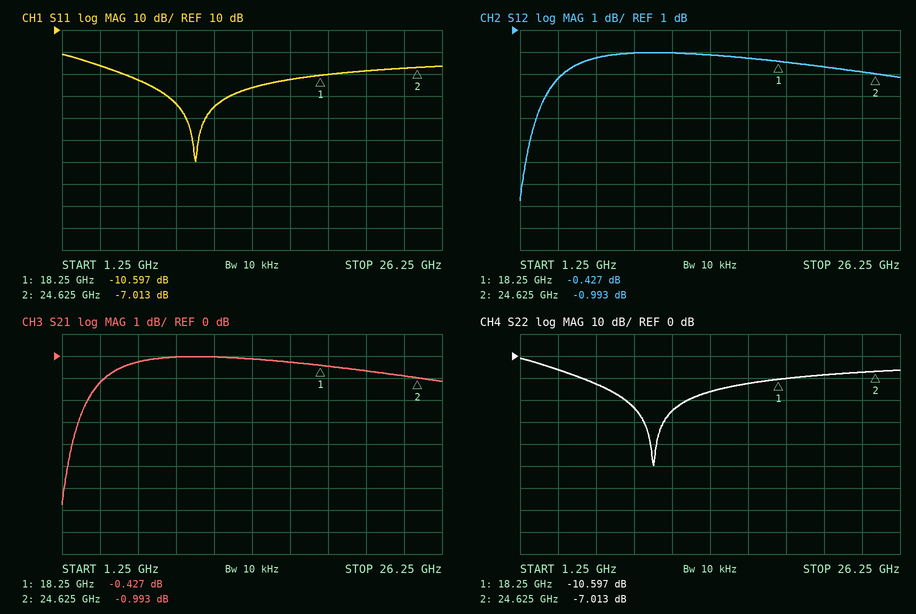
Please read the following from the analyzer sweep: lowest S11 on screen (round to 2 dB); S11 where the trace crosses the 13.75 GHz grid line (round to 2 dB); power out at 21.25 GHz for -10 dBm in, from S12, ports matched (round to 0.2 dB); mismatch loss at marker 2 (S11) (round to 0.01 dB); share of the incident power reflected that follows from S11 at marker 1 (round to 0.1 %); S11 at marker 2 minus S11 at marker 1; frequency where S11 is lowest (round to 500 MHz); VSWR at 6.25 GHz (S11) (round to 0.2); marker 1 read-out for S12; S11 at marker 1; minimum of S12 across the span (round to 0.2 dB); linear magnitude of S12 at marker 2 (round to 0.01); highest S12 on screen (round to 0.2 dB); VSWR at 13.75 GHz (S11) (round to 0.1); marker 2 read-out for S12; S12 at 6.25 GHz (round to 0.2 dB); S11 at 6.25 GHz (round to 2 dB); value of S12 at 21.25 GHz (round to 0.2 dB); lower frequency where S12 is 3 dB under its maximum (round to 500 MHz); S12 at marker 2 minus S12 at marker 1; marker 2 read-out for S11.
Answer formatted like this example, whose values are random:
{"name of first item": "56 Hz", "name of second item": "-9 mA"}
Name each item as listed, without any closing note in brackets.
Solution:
{"lowest S11 on screen": "-50 dB", "S11 where the trace crosses the 13.75 GHz grid line": "-16 dB", "power out at 21.25 GHz for -10 dBm in, from S12, ports matched": "-10.6 dBm", "mismatch loss at marker 2 (S11)": "0.96 dB", "share of the incident power reflected that follows from S11 at marker 1": "8.7 %", "S11 at marker 2 minus S11 at marker 1": "3.584 dB", "frequency where S11 is lowest": "10.0 GHz", "VSWR at 6.25 GHz (S11)": "1.6", "marker 1 read-out for S12": "-0.427 dB", "S11 at marker 1": "-10.597 dB", "minimum of S12 across the span": "-6.8 dB", "linear magnitude of S12 at marker 2": "0.89", "highest S12 on screen": "0.0 dB", "VSWR at 13.75 GHz (S11)": "1.4", "marker 2 read-out for S12": "-0.993 dB", "S12 at 6.25 GHz": "-0.2 dB", "S11 at 6.25 GHz": "-12 dB", "value of S12 at 21.25 GHz": "-0.6 dB", "lower frequency where S12 is 3 dB under its maximum": "2.5 GHz", "S12 at marker 2 minus S12 at marker 1": "-0.566 dB", "marker 2 read-out for S11": "-7.013 dB"}
